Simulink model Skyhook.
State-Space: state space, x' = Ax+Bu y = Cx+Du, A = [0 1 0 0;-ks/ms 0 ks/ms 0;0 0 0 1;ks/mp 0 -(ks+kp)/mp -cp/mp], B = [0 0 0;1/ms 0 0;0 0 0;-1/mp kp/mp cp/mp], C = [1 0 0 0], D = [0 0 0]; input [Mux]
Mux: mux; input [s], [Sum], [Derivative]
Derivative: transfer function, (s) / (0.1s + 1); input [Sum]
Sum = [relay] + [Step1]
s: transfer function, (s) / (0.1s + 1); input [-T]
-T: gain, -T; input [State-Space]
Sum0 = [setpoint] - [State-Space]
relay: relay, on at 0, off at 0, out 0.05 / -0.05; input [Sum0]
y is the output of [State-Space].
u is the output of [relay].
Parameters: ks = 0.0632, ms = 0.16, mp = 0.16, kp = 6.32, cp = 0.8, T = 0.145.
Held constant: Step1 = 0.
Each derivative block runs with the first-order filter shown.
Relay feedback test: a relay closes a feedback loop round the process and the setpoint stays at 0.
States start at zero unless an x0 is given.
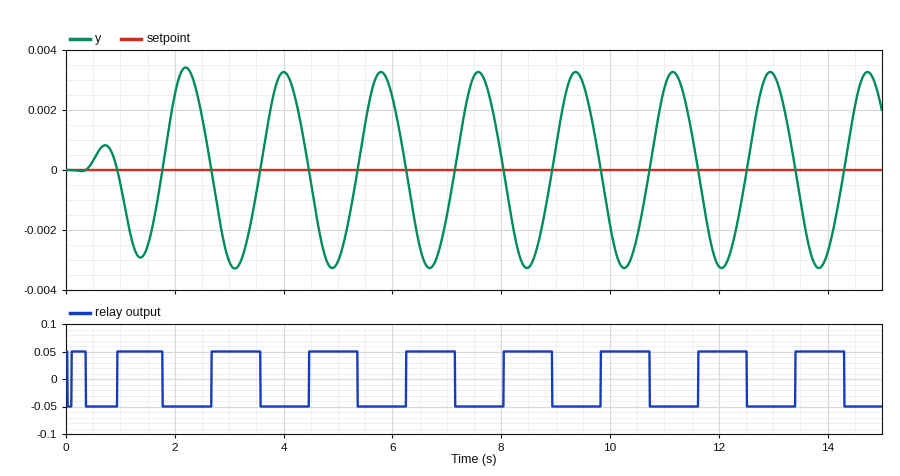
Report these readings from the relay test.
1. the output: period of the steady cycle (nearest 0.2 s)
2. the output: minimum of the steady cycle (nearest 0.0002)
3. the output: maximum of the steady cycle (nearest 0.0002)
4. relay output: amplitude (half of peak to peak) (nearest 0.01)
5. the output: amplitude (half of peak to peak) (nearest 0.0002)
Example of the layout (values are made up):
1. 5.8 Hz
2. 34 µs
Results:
1. 1.8 s
2. -0.0032
3. 0.0032
4. 0.05
5. 0.0032
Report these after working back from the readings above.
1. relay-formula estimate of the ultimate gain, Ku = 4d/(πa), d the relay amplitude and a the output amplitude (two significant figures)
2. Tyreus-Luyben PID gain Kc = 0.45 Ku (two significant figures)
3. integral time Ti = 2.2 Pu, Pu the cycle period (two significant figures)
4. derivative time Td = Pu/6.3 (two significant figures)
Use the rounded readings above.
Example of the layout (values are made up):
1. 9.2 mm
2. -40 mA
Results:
1. 20
2. 9.0
3. 4.0 s
4. 0.29 s
